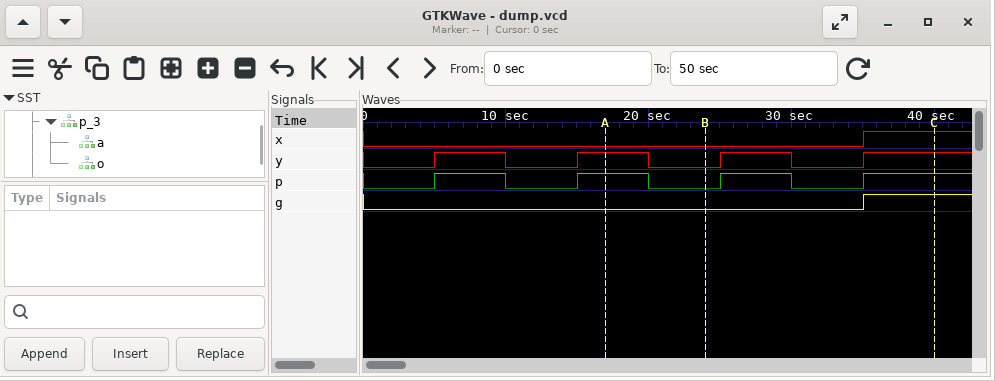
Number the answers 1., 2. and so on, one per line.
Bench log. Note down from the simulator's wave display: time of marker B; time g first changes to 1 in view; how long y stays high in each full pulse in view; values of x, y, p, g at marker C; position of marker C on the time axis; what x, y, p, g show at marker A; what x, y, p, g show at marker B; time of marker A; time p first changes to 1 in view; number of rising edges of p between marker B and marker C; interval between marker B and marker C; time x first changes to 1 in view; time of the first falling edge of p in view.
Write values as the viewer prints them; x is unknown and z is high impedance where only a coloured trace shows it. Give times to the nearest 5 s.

1. 25 s
2. 35 s
3. 5 s, 5 s, 5 s
4. x=1, y=1, p=1, g=1
5. 40 s
6. x=0, y=1, p=1, g=0
7. x=0, y=0, p=0, g=0
8. 15 s
9. 5 s
10. 2
11. 15 s
12. 35 s
13. 10 s
